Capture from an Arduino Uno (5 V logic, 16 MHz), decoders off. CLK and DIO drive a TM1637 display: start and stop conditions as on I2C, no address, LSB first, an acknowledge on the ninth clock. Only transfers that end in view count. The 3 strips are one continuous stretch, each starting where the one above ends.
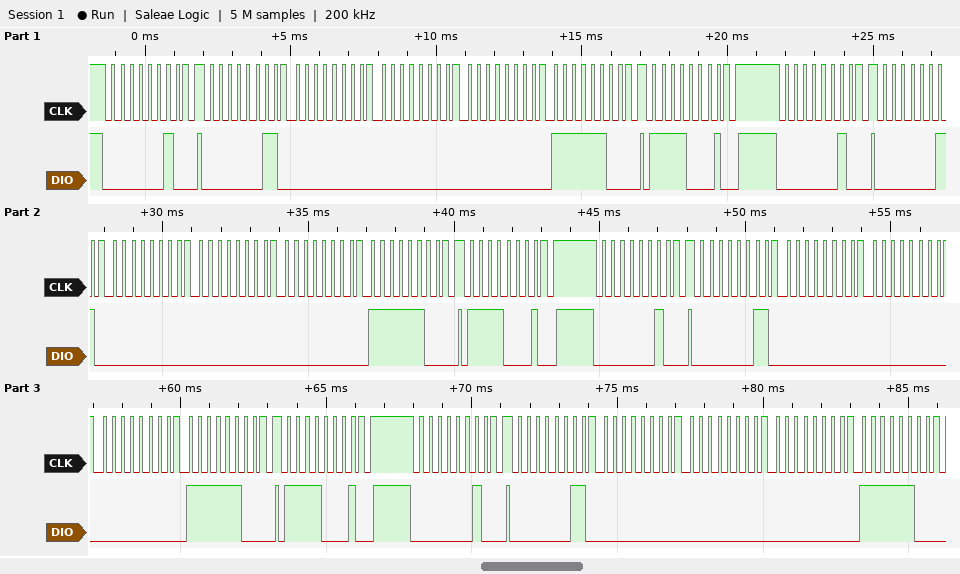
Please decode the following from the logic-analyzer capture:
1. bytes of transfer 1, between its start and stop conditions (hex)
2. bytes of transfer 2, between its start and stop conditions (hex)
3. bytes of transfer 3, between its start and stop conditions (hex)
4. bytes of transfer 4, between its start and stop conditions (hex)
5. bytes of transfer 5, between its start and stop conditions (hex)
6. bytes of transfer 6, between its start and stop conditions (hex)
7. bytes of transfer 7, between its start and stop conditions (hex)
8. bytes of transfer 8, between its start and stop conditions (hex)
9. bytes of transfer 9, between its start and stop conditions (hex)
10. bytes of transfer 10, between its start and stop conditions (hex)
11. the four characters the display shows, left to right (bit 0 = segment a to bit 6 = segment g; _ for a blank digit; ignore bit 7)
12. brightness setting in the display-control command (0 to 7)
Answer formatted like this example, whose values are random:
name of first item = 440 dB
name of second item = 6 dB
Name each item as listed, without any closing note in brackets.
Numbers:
bytes of transfer 1, between its start and stop conditions = 40
bytes of transfer 2, between its start and stop conditions = C0 00 00 00 3F
bytes of transfer 3, between its start and stop conditions = 8F
bytes of transfer 4, between its start and stop conditions = 40
bytes of transfer 5, between its start and stop conditions = C0 00 00 00 3F
bytes of transfer 6, between its start and stop conditions = 8F
bytes of transfer 7, between its start and stop conditions = 40
bytes of transfer 8, between its start and stop conditions = C0 00 00 00 3F
bytes of transfer 9, between its start and stop conditions = 8F
bytes of transfer 10, between its start and stop conditions = 40
the four characters the display shows, left to right = ___0
brightness setting in the display-control command = 7
